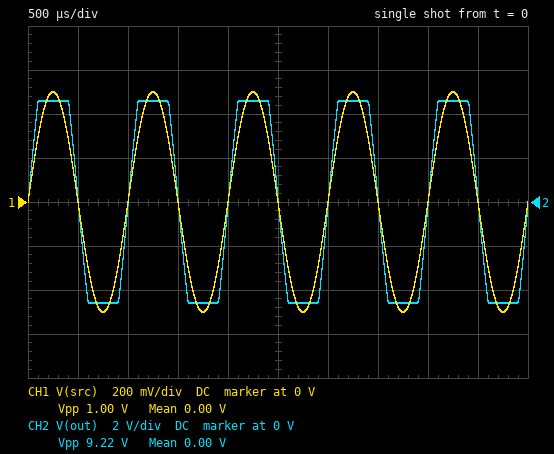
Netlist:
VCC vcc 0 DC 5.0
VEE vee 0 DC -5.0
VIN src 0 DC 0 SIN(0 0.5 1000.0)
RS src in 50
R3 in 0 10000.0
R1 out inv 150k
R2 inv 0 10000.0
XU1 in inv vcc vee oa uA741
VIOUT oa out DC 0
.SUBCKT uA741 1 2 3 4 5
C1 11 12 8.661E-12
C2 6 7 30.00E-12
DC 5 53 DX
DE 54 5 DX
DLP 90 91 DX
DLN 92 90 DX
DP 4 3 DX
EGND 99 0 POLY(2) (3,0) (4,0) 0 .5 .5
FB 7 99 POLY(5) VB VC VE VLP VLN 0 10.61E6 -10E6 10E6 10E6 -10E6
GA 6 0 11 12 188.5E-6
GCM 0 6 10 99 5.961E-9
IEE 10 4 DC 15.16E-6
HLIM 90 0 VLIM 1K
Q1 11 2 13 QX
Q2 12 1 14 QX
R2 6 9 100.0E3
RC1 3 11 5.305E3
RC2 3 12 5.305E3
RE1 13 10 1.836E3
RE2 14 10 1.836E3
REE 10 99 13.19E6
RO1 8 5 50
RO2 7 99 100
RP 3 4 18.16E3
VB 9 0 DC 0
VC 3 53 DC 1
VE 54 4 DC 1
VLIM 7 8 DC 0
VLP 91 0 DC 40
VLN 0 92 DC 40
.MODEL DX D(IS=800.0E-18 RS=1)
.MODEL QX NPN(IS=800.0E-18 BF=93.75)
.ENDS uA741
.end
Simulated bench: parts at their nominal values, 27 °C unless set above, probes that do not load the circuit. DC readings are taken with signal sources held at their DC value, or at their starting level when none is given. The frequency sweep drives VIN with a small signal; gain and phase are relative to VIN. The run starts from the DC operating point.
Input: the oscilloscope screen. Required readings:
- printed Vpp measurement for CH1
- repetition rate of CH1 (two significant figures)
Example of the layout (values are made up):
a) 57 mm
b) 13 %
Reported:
a) 1.00 V
b) 1.0 kHz
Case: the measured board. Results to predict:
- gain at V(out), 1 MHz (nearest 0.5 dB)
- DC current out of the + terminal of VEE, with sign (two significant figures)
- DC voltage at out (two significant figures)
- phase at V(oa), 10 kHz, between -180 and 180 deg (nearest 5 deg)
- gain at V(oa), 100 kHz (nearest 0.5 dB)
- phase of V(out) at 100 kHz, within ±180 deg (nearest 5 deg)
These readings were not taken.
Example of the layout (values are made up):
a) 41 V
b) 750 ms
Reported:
a) -1.0 dB
b) -570 µA
c) 12 mV
d) -10 deg
e) 18.5 dB
f) -60 deg
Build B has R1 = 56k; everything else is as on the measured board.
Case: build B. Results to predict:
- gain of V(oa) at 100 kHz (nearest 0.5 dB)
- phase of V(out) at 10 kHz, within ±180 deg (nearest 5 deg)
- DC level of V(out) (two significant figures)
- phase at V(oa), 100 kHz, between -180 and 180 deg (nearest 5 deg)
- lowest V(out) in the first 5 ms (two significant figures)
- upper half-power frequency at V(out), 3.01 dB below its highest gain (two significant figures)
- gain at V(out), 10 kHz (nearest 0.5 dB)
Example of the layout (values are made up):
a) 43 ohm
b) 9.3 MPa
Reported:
a) 15.0 dB
b) -5 deg
c) 4.6 mV
d) -35 deg
e) -3.3 V
f) 160 kHz
g) 16.5 dB
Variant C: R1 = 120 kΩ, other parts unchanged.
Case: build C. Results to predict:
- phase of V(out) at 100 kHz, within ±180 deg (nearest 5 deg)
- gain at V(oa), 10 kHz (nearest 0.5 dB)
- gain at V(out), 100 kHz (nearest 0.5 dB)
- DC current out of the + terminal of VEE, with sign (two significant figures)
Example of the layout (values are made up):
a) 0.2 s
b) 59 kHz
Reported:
a) -55 deg
b) 22.0 dB
c) 18.0 dB
d) -570 µA
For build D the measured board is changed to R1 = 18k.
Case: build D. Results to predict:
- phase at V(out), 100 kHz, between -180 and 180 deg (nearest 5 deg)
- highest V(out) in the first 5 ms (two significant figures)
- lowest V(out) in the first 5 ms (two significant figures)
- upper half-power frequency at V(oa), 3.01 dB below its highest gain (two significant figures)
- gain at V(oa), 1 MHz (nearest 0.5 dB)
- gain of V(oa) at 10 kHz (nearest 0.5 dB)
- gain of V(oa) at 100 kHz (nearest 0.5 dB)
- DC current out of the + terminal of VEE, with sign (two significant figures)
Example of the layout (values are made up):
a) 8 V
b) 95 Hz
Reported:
a) -15 deg
b) 1.4 V
c) -1.4 V
d) 440 kHz
e) -0.5 dB
f) 9.0 dB
g) 8.5 dB
h) -570 µA
